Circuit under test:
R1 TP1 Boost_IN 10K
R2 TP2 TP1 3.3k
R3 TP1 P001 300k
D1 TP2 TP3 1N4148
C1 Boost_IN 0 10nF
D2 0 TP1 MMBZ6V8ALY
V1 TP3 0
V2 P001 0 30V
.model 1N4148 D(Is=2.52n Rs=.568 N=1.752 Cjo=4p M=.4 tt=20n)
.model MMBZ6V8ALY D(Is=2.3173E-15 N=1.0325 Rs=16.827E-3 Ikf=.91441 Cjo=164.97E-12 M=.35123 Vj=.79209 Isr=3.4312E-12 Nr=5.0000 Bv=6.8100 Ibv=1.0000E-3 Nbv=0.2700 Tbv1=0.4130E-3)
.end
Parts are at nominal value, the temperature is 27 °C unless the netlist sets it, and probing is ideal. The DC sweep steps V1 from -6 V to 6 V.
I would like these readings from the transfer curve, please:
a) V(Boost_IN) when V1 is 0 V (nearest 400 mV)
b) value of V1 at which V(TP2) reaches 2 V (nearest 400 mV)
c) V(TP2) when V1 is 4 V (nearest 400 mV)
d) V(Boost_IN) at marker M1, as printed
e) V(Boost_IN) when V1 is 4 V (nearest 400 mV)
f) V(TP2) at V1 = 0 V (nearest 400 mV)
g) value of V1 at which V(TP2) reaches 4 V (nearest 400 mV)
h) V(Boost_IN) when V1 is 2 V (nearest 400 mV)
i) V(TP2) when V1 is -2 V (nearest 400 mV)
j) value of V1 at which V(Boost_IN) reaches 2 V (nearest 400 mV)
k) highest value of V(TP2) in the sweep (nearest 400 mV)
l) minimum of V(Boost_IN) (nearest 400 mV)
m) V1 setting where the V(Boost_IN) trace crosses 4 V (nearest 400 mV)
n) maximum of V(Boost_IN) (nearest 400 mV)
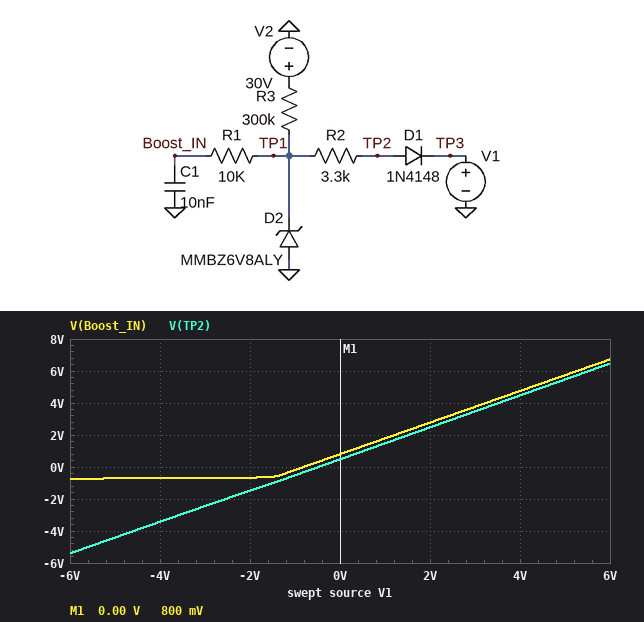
800 mV
1.6 V
4.4 V
800 mV
4.8 V
400 mV
3.6 V
2.8 V
-1.6 V
1.2 V
6.4 V
-800 mV
3.2 V
6.8 V
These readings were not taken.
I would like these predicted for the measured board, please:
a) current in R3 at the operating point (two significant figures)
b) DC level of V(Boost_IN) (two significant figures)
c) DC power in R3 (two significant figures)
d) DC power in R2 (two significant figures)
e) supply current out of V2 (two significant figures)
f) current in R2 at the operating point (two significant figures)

97 µA
800 mV
2.8 mW
31 µW
97 µA
97 µA
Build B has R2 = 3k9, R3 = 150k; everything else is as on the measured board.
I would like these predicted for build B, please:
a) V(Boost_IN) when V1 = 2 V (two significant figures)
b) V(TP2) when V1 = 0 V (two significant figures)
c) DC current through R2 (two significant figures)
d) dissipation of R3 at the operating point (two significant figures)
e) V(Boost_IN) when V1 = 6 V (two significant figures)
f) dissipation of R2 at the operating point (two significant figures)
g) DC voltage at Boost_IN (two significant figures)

3.2 V
510 mV
190 µA
5.5 mW
6.8 V
140 µW
1.3 V
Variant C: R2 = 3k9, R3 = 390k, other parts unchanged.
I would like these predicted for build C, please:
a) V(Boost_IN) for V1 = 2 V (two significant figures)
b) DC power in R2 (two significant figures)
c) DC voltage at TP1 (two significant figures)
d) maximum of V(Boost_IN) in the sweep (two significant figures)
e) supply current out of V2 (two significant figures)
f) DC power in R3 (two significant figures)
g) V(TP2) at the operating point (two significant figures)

2.7 V
22 µW
760 mV
6.7 V
75 µA
2.2 mW
470 mV
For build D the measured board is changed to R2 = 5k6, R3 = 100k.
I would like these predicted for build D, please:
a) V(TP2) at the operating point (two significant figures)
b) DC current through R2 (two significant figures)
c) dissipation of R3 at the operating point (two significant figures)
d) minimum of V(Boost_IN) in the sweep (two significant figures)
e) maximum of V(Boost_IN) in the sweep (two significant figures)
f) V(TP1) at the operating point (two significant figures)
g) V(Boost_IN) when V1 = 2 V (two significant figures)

530 mV
280 µA
7.8 mW
-700 mV
6.8 V
2.1 V
4.0 V
